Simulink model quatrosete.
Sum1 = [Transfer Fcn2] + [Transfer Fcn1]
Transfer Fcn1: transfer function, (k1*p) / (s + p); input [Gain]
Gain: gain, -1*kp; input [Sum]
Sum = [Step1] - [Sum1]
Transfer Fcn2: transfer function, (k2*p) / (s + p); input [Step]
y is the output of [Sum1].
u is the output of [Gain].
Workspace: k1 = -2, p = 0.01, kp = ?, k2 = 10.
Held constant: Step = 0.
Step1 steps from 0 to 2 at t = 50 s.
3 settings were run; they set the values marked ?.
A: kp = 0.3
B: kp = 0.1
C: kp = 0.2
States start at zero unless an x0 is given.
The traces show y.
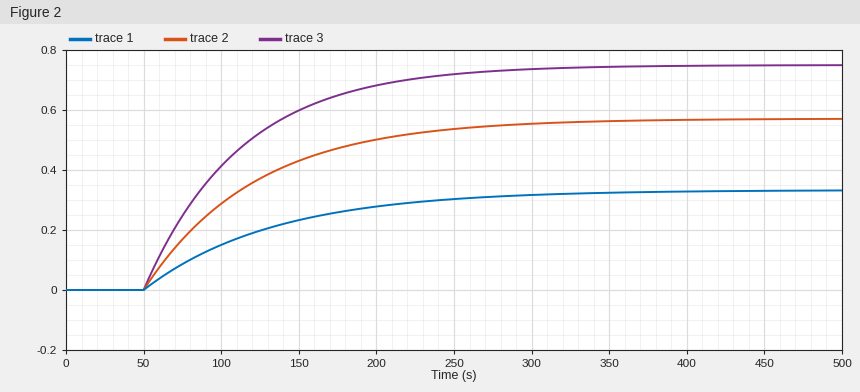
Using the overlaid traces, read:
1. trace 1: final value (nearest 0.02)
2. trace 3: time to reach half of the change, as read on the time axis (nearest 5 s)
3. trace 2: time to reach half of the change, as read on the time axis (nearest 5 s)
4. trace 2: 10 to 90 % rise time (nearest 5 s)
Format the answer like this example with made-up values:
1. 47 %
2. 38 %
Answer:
1. 0.34
2. 95 s
3. 100 s
4. 155 s
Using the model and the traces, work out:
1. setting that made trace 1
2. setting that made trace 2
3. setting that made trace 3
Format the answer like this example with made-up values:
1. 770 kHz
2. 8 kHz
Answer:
1. B
2. C
3. A
